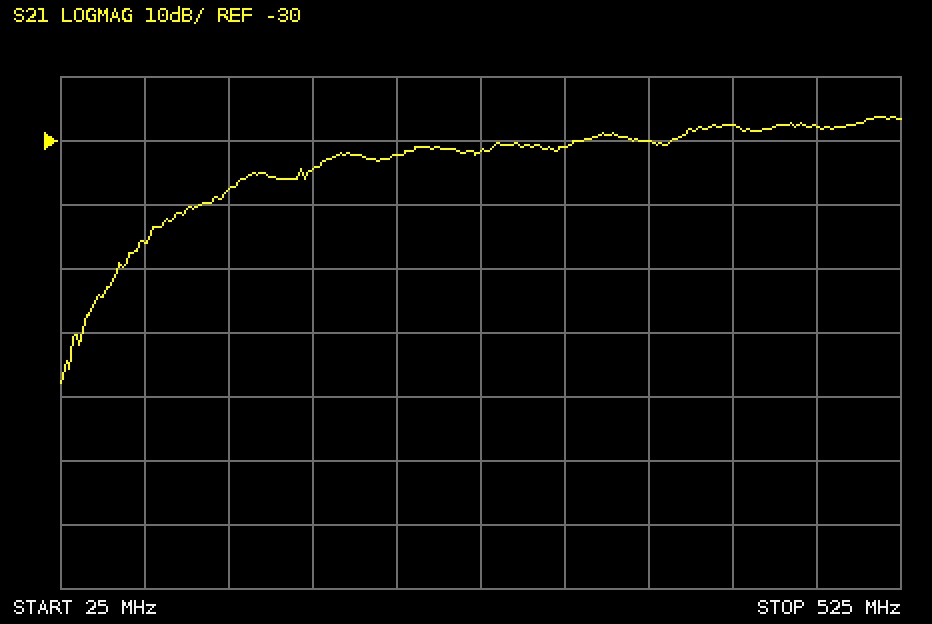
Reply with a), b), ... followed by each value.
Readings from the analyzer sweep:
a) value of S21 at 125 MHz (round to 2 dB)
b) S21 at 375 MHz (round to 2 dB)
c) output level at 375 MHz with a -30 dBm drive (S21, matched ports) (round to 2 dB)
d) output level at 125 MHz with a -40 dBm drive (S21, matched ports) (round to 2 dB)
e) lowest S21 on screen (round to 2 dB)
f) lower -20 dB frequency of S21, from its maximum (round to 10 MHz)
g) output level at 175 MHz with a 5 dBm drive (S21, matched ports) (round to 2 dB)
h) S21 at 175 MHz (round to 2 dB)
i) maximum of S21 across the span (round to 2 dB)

a) -38 dB
b) -30 dB
c) -60 dBm
d) -78 dBm
e) -68 dB
f) 70 MHz
g) -30 dBm
h) -34 dB
i) -26 dB
